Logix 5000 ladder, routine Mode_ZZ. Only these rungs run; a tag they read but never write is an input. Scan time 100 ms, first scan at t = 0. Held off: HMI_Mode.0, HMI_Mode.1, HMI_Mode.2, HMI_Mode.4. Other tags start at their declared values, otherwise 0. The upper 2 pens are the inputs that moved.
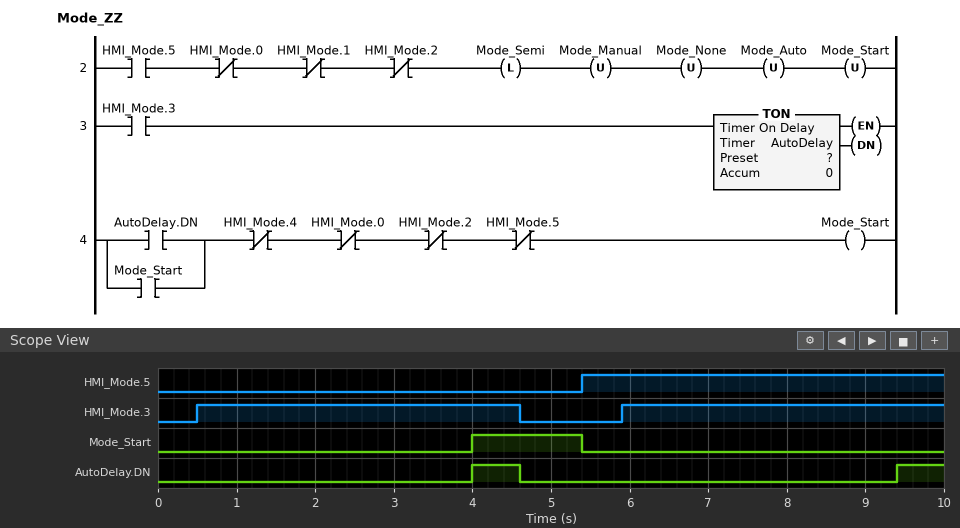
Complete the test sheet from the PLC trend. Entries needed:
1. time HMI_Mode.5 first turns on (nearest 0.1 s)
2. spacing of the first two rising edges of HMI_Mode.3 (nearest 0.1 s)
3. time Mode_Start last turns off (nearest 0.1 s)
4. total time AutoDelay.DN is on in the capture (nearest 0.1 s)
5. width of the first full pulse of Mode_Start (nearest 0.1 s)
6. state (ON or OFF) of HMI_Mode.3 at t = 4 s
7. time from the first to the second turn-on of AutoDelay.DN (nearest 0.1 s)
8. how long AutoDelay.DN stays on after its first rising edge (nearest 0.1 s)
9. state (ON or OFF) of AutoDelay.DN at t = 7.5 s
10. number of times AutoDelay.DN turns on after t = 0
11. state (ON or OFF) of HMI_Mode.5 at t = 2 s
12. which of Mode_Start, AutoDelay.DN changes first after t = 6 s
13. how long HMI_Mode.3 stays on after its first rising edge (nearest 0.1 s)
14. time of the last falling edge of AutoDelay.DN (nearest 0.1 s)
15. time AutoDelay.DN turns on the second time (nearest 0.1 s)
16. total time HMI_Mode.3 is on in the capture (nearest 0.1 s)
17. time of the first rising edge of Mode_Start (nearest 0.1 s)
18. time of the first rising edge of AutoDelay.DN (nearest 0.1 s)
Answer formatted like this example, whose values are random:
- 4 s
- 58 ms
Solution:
- 5.4 s
- 5.4 s
- 5.4 s
- 1.2 s
- 1.4 s
- ON
- 5.4 s
- 0.6 s
- OFF
- 2
- OFF
- AutoDelay.DN
- 4.1 s
- 4.6 s
- 9.4 s
- 8.2 s
- 4.0 s
- 4.0 s
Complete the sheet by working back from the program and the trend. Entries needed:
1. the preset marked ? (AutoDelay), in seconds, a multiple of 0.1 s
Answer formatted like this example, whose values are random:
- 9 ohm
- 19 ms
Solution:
- 3.5 s
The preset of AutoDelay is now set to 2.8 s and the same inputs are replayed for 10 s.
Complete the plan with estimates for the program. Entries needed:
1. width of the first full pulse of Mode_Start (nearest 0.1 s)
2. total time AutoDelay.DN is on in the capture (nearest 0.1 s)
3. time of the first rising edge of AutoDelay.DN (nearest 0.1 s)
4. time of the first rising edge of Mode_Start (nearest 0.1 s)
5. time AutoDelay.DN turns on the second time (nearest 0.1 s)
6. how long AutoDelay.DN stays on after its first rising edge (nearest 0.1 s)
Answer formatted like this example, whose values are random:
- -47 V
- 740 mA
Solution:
- 2.1 s
- 2.6 s
- 3.3 s
- 3.3 s
- 8.7 s
- 1.3 s
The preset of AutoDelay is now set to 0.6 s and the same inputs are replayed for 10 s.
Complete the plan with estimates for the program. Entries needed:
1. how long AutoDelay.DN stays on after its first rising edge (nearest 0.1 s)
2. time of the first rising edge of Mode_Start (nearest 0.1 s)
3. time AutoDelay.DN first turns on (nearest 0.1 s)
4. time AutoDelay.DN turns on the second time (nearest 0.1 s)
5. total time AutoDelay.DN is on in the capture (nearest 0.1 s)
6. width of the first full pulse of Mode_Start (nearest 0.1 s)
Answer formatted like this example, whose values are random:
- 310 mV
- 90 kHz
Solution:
- 3.5 s
- 1.1 s
- 1.1 s
- 6.5 s
- 7.0 s
- 4.3 s
